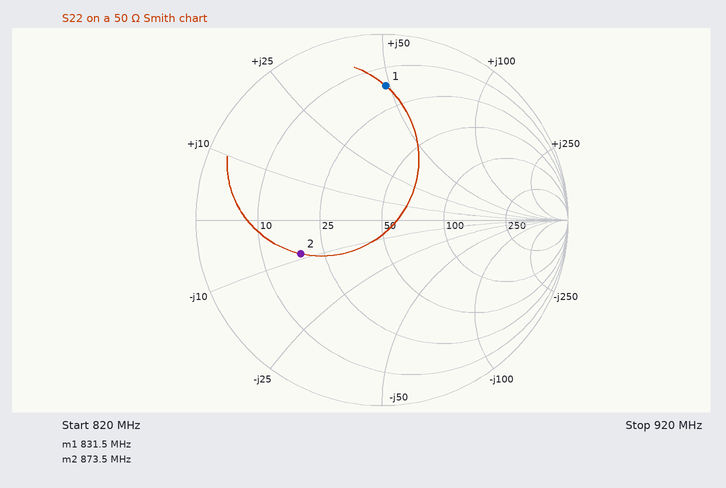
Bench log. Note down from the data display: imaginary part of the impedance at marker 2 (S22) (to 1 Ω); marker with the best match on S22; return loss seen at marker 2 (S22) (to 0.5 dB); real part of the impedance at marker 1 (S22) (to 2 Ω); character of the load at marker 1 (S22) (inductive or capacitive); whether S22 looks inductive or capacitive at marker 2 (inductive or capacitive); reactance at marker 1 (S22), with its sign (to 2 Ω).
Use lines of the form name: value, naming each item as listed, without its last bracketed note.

imaginary part of the impedance at marker 2 (S22): -9 Ω
marker with the best match on S22: marker 2
return loss seen at marker 2 (S22): 6.5 dB
real part of the impedance at marker 1 (S22): 16 Ω
character of the load at marker 1 (S22): inductive
whether S22 looks inductive or capacitive at marker 2: capacitive
reactance at marker 1 (S22), with its sign: +48 Ω
